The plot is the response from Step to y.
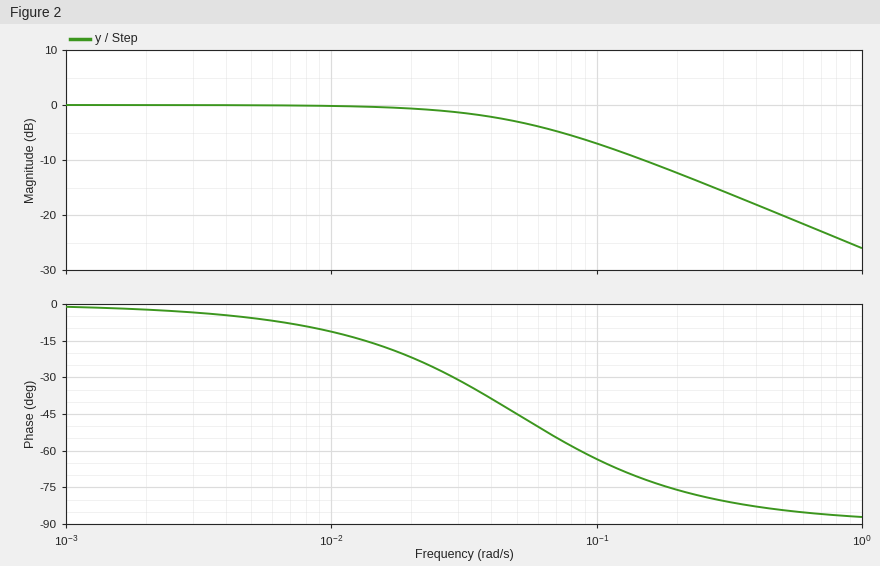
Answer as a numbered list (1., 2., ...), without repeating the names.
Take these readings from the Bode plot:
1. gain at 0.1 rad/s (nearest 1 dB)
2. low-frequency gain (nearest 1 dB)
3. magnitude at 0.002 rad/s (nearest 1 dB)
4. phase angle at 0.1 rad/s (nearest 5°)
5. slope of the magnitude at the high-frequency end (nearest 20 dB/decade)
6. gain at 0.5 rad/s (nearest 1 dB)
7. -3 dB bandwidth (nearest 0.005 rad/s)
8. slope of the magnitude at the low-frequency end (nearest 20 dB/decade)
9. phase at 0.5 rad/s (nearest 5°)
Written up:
1. -7 dB
2. 0 dB
3. 0 dB
4. -65°
5. -20 dB/decade
6. -20 dB
7. 0.050 rad/s
8. 0 dB/decade
9. -85°
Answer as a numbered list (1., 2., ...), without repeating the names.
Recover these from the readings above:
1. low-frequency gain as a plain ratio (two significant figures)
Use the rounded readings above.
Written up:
1. 1.0
